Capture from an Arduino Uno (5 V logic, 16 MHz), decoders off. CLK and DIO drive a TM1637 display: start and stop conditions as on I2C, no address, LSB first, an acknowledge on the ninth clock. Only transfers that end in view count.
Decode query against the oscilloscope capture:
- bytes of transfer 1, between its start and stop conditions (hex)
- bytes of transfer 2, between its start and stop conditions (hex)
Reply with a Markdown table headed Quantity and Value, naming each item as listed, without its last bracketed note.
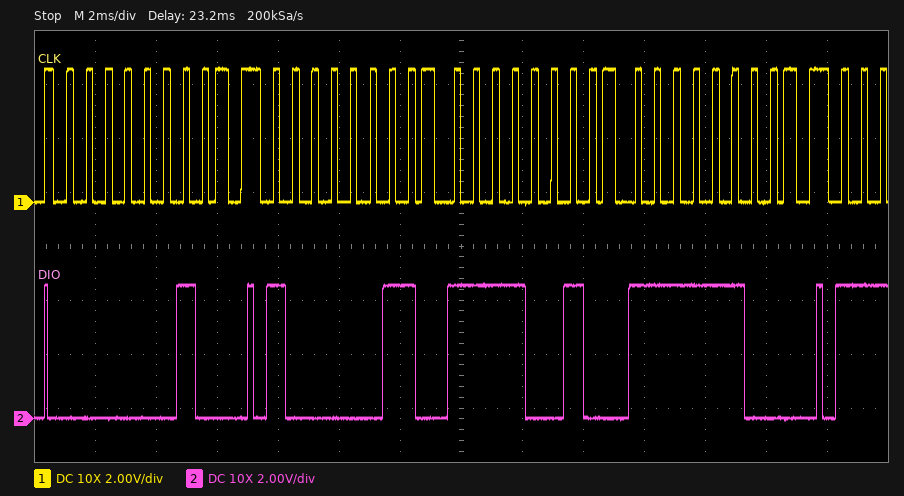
| Quantity | Value |
|---|---|
| bytes of transfer 1, between its start and stop conditions | 40 |
| bytes of transfer 2, between its start and stop conditions | C1 4F 3F |
